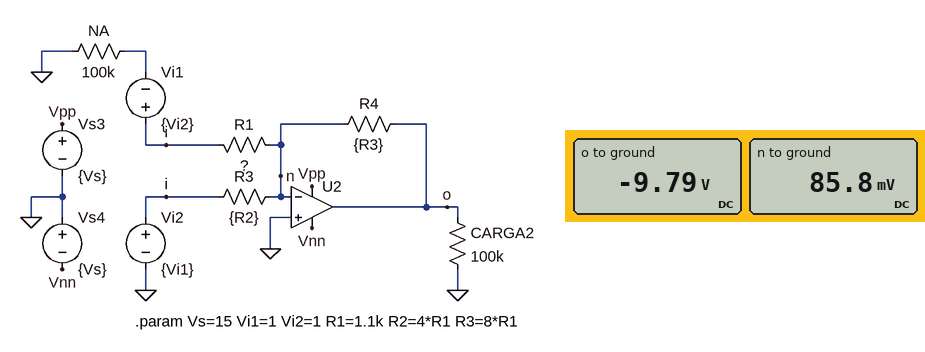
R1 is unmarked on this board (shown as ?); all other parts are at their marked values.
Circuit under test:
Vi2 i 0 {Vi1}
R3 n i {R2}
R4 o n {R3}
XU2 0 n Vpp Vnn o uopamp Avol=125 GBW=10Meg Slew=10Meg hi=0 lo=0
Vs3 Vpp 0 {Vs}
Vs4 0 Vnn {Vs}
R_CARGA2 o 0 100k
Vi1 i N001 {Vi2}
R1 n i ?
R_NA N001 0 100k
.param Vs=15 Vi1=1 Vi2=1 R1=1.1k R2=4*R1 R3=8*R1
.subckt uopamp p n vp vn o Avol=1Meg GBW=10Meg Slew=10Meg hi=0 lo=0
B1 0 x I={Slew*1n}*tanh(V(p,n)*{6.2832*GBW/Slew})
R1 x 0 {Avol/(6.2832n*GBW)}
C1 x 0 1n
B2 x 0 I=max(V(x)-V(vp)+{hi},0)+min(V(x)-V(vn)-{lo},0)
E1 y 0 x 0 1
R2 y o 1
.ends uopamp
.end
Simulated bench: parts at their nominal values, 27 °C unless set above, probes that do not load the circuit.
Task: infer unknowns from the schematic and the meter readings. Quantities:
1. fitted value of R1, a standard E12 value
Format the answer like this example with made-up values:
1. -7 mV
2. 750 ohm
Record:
1. 1 kΩ
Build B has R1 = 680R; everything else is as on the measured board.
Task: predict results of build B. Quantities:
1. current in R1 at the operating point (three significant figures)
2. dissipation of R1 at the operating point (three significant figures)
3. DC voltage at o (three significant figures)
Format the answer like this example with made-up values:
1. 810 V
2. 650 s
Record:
1. 1.29 mA
2. 1.13 mW
3. -13.0 V
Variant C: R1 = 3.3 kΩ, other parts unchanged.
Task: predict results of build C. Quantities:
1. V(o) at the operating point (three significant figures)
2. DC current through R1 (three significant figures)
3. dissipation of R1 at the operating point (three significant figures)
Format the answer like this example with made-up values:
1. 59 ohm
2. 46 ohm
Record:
1. -4.46 V
2. 292 µA
3. 281 µW
